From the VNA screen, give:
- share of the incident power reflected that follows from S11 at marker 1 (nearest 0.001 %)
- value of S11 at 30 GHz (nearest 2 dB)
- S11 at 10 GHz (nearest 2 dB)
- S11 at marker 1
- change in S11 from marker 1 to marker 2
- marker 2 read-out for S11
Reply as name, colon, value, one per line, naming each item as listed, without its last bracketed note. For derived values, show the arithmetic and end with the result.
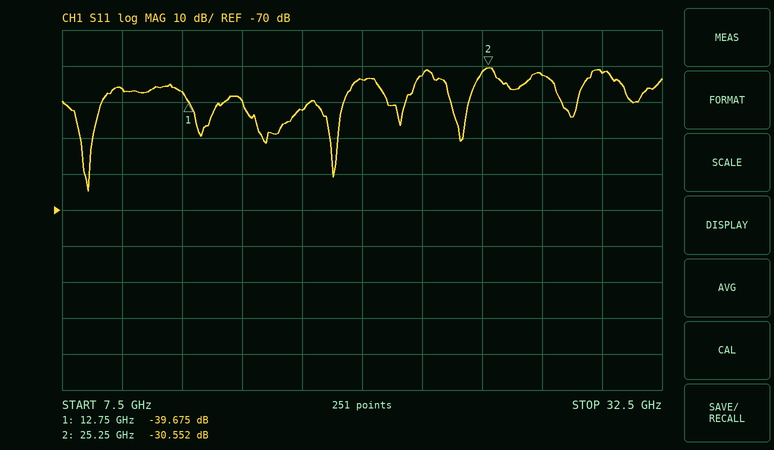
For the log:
share of the incident power reflected that follows from S11 at marker 1: 10^(-39.675/10) ≈ 0.011 %
value of S11 at 30 GHz: -32 dB
S11 at 10 GHz: -36 dB
S11 at marker 1: -39.675 dB
change in S11 from marker 1 to marker 2: -30.552 − (-39.675) = 9.123 dB
marker 2 read-out for S11: -30.552 dB
